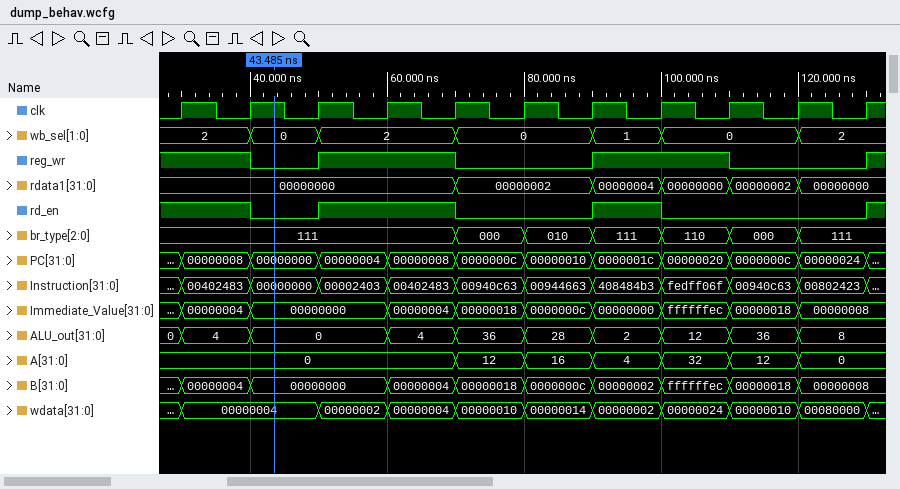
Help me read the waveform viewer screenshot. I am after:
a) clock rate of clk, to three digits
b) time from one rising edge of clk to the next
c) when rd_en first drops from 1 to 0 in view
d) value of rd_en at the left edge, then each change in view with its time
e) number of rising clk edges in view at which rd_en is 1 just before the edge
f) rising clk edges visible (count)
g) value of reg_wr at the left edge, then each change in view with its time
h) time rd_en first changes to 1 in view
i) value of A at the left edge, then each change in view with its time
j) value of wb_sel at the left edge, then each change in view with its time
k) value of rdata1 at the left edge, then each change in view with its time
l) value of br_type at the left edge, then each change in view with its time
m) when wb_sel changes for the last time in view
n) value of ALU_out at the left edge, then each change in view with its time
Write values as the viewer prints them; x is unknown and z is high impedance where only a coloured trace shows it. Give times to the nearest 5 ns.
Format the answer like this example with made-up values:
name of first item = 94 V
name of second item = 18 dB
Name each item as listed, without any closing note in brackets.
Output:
clock rate of clk, to three digits = 100 MHz
time from one rising edge of clk to the next = 10 ns
when rd_en first drops from 1 to 0 in view = 40 ns
value of rd_en at the left edge, then each change in view with its time = 1, 0 at 40 ns, 1 at 50 ns, 0 at 70 ns, 1 at 90 ns, 0 at 100 ns, 1 at 130 ns
number of rising clk edges in view at which rd_en is 1 just before the edge = 5
rising clk edges visible = 11
value of reg_wr at the left edge, then each change in view with its time = 1, 0 at 40 ns, 1 at 50 ns, 0 at 70 ns, 1 at 90 ns, 0 at 110 ns, 1 at 130 ns
time rd_en first changes to 1 in view = 50 ns
value of A at the left edge, then each change in view with its time = 0, 12 at 70 ns, 16 at 80 ns, 4 at 90 ns, 32 at 100 ns, 12 at 110 ns, 0 at 120 ns
value of wb_sel at the left edge, then each change in view with its time = 2, 0 at 40 ns, 2 at 50 ns, 0 at 70 ns, 1 at 90 ns, 0 at 100 ns, 2 at 120 ns
value of rdata1 at the left edge, then each change in view with its time = 00000000, 00000002 at 70 ns, 00000004 at 90 ns, 00000000 at 100 ns, 00000002 at 110 ns, 00000000 at 120 ns
value of br_type at the left edge, then each change in view with its time = 111, 000 at 70 ns, 010 at 80 ns, 111 at 90 ns, 110 at 100 ns, 000 at 110 ns, 111 at 120 ns
when wb_sel changes for the last time in view = 120 ns
value of ALU_out at the left edge, then each change in view with its time = 0, 4 at 30 ns, 0 at 40 ns, 4 at 60 ns, 36 at 70 ns, 28 at 80 ns, 2 at 90 ns, 12 at 100 ns, 36 at 110 ns, 8 at 120 ns
